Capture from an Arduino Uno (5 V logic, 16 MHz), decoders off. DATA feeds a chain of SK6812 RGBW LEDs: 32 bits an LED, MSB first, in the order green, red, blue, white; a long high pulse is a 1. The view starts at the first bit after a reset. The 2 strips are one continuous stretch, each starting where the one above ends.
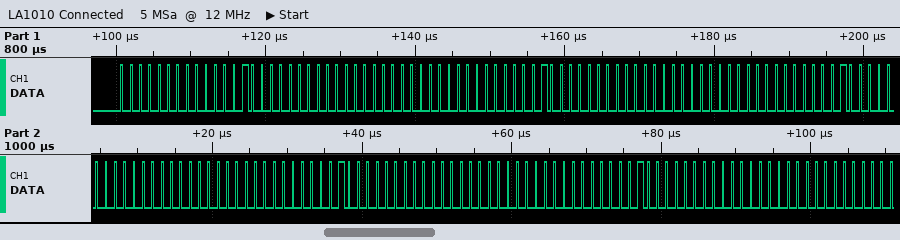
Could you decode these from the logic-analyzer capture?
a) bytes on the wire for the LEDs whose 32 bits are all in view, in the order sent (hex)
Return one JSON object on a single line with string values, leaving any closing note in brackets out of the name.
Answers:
{"bytes on the wire for the LEDs whose 32 bits are all in view, in the order sent": "00 04 00 00 00 04 00 00 00 04 00 00 00 04 00 00 00 04 00 00"}
